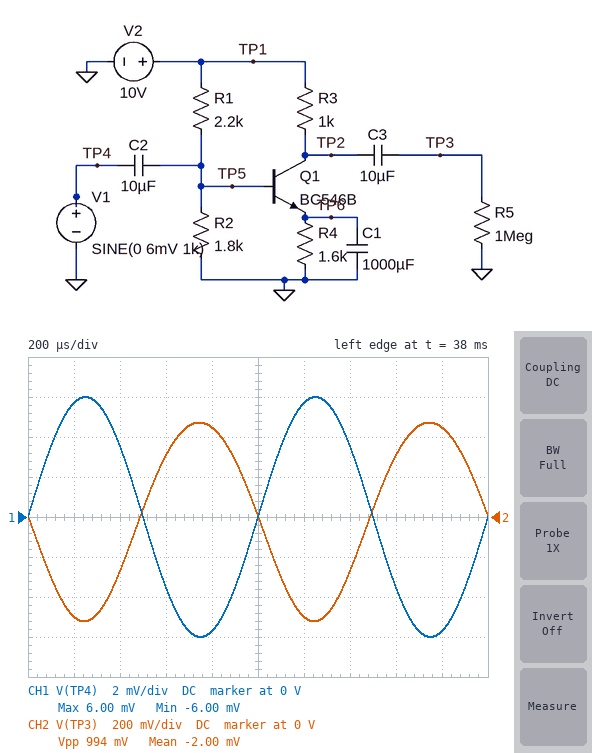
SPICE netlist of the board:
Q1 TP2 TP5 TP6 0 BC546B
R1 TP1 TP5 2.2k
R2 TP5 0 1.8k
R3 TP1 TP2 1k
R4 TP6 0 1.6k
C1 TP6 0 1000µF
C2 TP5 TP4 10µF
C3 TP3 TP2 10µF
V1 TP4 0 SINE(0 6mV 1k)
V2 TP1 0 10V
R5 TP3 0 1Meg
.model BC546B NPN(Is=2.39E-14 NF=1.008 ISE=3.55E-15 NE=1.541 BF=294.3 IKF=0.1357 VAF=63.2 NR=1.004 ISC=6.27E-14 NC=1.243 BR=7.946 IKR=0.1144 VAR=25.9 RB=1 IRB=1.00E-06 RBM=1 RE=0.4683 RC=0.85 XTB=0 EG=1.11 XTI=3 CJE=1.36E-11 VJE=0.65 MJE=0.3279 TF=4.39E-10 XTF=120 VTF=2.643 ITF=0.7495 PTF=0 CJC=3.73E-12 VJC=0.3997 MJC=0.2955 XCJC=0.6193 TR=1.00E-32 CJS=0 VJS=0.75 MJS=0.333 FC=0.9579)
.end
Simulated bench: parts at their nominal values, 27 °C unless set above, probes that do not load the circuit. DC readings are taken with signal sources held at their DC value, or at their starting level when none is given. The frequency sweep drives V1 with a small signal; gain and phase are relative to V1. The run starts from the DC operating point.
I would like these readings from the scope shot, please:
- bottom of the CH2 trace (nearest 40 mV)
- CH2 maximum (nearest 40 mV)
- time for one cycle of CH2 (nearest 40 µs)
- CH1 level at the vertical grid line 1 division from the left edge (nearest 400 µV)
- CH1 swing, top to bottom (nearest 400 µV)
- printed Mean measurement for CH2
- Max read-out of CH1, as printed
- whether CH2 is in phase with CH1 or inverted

-520 mV
480 mV
1.00 ms
5.6 mV
12.0 mV
-2.00 mV
6.00 mV
inverted
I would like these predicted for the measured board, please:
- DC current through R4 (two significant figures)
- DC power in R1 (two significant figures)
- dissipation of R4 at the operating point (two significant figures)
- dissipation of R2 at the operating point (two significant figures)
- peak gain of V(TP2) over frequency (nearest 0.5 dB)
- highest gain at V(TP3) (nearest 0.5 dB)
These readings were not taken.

2.4 mA
14 mW
9.2 mW
11 mW
38.5 dB
38.5 dB
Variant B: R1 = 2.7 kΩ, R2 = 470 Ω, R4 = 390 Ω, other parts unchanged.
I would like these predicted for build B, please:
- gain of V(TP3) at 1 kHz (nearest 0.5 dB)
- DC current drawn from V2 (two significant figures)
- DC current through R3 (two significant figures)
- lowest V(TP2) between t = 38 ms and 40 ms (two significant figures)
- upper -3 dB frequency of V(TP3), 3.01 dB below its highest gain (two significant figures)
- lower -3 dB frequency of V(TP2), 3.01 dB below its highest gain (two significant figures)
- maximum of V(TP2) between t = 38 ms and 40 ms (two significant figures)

37.5 dB
5.3 mA
2.1 mA
7.4 V
96 MHz
48 Hz
8.3 V
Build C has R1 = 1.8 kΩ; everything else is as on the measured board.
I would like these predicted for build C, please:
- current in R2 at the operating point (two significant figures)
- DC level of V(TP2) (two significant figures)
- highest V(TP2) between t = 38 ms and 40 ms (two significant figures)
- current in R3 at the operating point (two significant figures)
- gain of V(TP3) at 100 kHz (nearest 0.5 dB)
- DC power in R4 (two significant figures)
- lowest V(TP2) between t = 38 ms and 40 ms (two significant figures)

2.8 mA
7.3 V
7.8 V
2.7 mA
39.5 dB
12 mW
6.7 V
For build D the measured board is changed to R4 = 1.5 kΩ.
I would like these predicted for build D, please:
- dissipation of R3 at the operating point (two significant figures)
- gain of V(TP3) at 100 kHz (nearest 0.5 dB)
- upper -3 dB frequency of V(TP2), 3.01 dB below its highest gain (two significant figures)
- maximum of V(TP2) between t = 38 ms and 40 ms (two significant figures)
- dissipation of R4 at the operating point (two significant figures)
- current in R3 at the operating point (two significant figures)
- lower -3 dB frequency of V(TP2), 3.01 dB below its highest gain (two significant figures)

6.5 mW
39.0 dB
78 MHz
8.0 V
9.8 mW
2.5 mA
29 Hz
